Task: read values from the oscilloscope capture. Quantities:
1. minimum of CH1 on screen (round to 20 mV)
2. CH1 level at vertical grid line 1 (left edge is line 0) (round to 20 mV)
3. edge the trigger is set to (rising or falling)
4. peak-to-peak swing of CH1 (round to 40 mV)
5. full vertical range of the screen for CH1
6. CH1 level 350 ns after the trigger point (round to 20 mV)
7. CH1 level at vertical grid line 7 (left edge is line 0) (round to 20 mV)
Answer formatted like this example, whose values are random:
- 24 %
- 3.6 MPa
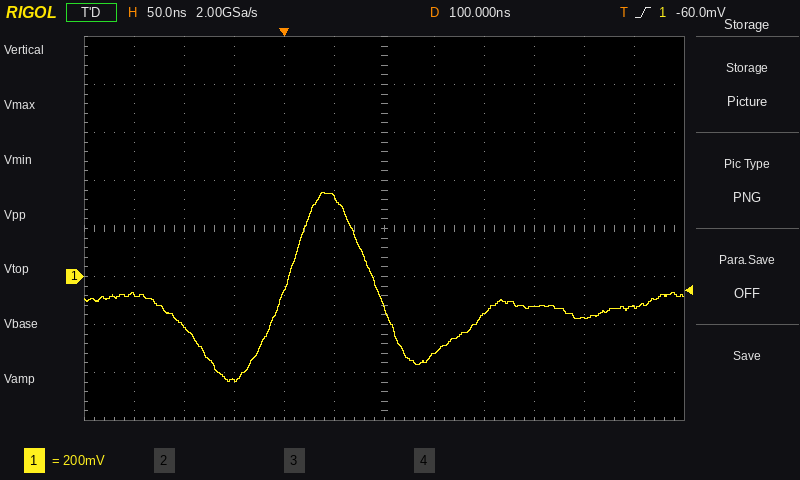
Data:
- -440 mV
- -80 mV
- rising
- 800 mV
- 1.6 V
- -120 mV
- -320 mV
